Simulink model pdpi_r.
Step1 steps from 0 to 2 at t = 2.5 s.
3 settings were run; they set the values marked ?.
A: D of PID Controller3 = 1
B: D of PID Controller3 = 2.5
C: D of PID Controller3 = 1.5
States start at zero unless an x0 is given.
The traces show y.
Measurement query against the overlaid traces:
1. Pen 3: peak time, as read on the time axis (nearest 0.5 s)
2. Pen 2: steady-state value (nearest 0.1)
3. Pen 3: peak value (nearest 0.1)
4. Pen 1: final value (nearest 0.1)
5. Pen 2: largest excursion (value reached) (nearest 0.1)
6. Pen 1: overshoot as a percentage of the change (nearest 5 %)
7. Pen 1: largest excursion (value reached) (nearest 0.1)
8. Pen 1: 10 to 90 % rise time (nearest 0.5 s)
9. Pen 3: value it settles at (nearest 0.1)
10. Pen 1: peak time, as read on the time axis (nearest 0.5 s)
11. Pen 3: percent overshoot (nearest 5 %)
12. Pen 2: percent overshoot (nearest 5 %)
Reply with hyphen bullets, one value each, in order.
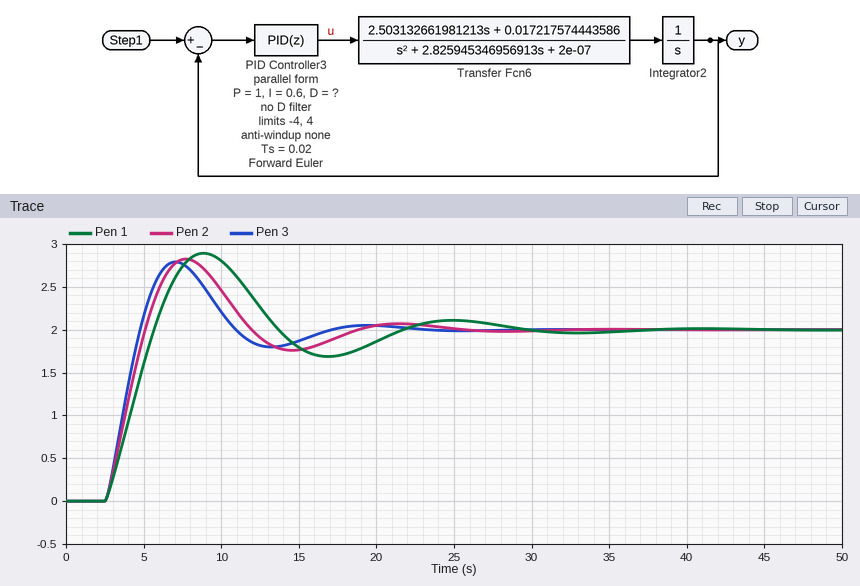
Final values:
- 7.0 s
- 2.0
- 2.8
- 2.0
- 2.8
- 45 %
- 2.9
- 2.5 s
- 2.0
- 9.0 s
- 40 %
- 40 %
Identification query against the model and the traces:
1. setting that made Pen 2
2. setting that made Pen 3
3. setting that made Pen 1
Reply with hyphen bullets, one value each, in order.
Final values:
- C
- A
- B
